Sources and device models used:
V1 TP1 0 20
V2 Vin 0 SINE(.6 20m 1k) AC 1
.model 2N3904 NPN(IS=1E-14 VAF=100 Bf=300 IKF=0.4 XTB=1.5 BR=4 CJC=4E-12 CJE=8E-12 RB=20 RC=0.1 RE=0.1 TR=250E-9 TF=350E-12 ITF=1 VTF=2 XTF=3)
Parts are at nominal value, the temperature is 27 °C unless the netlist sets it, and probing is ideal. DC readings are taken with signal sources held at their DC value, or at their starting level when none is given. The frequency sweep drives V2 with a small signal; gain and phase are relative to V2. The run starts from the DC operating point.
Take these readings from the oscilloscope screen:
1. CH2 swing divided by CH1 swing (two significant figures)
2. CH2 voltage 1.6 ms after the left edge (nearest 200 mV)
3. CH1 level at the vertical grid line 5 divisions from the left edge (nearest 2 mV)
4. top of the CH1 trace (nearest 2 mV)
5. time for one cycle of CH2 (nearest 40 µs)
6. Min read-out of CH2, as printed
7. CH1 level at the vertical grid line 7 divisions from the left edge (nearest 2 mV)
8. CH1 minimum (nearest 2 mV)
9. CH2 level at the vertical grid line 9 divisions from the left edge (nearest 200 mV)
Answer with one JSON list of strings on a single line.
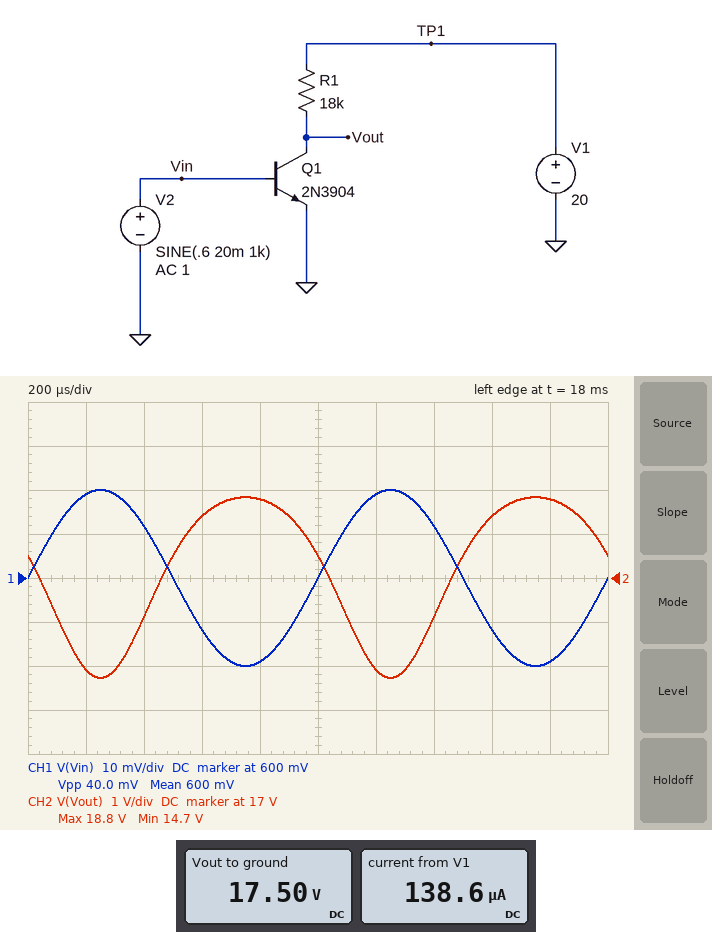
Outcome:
["100", "18.4 V", "600 mV", "620 mV", "1.00 ms", "14.7 V", "612 mV", "580 mV", "18.8 V"]
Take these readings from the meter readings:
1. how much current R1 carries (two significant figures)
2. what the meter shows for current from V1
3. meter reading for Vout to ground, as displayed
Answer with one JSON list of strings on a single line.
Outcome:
["140 µA", "138.6 µA", "17.50 V"]
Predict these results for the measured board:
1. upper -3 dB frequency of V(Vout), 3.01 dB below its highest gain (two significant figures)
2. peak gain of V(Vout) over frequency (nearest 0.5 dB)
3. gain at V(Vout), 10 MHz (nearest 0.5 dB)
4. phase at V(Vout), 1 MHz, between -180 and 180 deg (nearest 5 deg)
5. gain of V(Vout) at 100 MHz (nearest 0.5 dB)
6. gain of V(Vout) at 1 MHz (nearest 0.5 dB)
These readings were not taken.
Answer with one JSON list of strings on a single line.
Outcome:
["5.8 MHz", "39.5 dB", "33.5 dB", "170 deg", "14.5 dB", "39.5 dB"]
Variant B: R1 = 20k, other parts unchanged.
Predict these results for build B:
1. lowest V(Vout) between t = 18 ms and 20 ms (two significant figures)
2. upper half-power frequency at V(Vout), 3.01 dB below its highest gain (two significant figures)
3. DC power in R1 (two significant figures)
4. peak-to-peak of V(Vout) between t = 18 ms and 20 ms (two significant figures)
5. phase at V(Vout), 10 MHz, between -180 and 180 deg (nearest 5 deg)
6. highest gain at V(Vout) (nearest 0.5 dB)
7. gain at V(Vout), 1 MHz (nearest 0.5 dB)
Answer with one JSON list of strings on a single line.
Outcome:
["14 V", "5.2 MHz", "380 µW", "4.5 V", "115 deg", "40.5 dB", "40.0 dB"]
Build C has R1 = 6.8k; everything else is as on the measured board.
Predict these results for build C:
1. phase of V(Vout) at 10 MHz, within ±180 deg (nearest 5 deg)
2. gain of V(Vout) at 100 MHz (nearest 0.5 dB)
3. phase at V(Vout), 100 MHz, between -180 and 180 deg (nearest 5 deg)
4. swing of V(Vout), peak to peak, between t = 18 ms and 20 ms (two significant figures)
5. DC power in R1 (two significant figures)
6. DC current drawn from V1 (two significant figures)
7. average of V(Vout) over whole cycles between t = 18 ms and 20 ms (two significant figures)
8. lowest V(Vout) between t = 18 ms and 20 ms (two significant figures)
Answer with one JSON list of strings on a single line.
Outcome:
["145 deg", "15.0 dB", "80 deg", "1.6 V", "130 µW", "140 µA", "19 V", "18 V"]
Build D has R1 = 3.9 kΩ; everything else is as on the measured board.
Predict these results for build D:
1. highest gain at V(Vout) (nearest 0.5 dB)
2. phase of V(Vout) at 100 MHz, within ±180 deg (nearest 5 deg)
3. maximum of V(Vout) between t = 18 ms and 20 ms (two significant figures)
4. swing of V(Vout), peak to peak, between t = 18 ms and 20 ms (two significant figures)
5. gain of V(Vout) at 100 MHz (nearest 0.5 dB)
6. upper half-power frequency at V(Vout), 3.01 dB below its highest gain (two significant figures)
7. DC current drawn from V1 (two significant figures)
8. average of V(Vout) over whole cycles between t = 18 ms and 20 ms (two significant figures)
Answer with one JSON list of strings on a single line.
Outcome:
["26.5 dB", "85 deg", "20 V", "930 mV", "15.0 dB", "27 MHz", "140 µA", "19 V"]
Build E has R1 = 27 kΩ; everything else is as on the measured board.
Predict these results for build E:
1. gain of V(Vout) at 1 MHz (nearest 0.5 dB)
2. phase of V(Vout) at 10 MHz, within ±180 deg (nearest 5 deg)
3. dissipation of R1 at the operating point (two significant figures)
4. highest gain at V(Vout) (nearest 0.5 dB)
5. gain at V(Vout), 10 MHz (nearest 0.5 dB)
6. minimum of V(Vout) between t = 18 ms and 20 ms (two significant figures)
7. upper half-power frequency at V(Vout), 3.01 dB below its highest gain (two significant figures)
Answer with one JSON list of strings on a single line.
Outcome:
["42.5 dB", "110 deg", "510 µW", "43.0 dB", "34.0 dB", "12 V", "3.8 MHz"]
